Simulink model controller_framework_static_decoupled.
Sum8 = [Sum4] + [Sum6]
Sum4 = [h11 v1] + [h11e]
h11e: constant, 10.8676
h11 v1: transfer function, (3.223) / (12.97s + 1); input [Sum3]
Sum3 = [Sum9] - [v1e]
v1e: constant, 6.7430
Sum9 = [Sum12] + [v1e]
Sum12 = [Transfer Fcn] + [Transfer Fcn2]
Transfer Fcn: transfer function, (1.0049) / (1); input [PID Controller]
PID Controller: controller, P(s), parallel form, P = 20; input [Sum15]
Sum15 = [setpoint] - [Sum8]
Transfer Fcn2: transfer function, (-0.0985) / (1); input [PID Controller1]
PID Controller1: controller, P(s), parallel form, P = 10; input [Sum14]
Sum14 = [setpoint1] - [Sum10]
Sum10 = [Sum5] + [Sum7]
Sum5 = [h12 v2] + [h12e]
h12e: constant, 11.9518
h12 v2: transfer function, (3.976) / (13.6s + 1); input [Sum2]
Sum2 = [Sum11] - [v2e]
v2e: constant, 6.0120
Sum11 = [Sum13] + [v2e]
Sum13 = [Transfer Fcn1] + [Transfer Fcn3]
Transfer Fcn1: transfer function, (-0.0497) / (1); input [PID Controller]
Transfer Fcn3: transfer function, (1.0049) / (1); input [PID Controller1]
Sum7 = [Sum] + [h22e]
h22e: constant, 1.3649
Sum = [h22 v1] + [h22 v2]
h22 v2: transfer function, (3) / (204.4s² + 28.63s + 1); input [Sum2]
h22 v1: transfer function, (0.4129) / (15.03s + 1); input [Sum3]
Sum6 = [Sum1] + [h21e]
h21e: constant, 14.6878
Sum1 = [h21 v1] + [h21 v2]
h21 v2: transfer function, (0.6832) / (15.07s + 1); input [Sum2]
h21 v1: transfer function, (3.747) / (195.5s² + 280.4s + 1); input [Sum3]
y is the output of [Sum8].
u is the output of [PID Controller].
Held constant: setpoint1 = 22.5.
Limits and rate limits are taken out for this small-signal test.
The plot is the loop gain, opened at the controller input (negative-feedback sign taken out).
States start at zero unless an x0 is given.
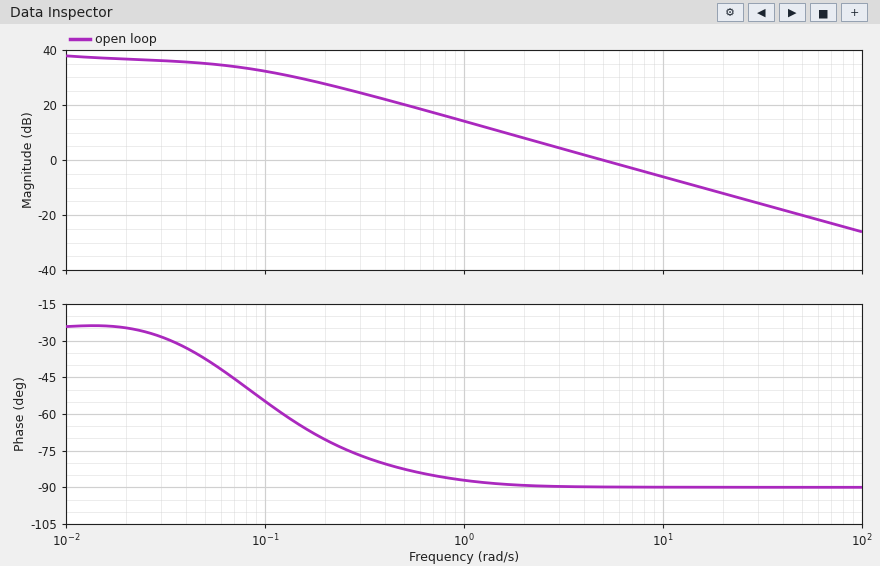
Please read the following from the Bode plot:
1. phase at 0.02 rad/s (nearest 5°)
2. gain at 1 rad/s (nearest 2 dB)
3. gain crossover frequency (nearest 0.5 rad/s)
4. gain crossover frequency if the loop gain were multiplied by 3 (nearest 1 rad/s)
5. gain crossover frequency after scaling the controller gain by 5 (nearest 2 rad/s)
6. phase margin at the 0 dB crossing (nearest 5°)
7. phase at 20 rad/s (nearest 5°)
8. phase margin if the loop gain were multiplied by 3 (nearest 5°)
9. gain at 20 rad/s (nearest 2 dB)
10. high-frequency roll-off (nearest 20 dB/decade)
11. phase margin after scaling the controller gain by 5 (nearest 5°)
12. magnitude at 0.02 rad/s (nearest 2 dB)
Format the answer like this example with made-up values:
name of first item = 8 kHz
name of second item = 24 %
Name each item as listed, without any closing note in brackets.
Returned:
phase at 0.02 rad/s = -25°
gain at 1 rad/s = 14 dB
gain crossover frequency = 5.0 rad/s
gain crossover frequency if the loop gain were multiplied by 3 = 15 rad/s
gain crossover frequency after scaling the controller gain by 5 = 24 rad/s
phase margin at the 0 dB crossing = 90°
phase at 20 rad/s = -90°
phase margin if the loop gain were multiplied by 3 = 90°
gain at 20 rad/s = -12 dB
high-frequency roll-off = -20 dB/decade
phase margin after scaling the controller gain by 5 = 90°
magnitude at 0.02 rad/s = 36 dB
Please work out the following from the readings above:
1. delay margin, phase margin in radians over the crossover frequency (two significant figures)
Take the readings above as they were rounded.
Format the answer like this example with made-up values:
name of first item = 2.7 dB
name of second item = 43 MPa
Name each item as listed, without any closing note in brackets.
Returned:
delay margin, phase margin in radians over the crossover frequency = 0.31 s
